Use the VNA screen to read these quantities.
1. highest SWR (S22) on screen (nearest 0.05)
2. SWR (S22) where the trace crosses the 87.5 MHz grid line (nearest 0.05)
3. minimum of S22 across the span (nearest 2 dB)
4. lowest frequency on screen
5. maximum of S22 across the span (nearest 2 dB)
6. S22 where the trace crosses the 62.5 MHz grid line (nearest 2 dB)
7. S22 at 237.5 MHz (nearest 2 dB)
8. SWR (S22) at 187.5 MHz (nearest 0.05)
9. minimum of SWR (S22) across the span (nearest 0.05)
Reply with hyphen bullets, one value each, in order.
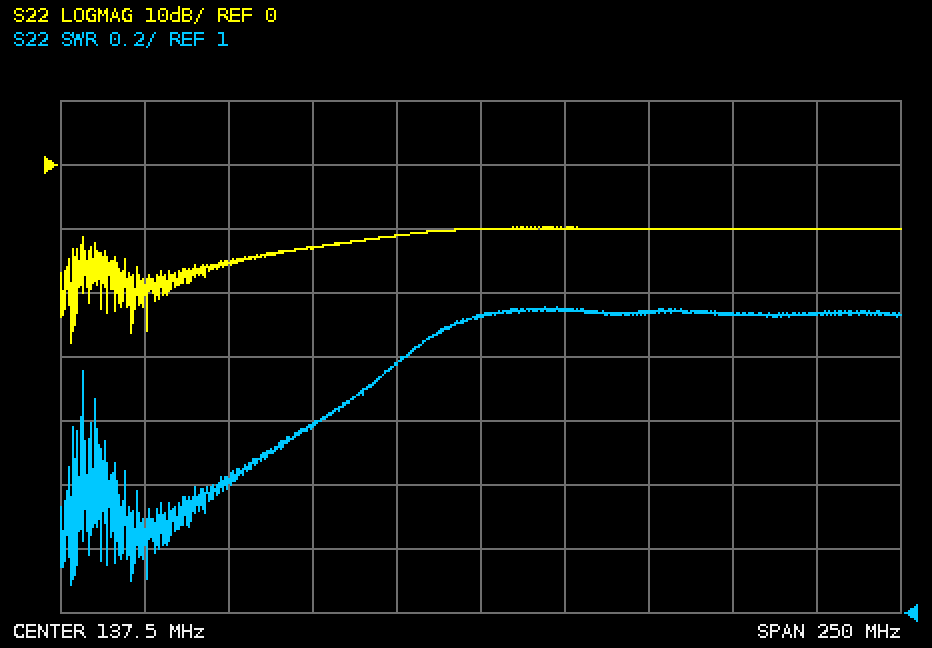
- 1.95
- 1.60
- -28 dB
- 12.5 MHz
- -10 dB
- -16 dB
- -10 dB
- 1.95
- 1.10
